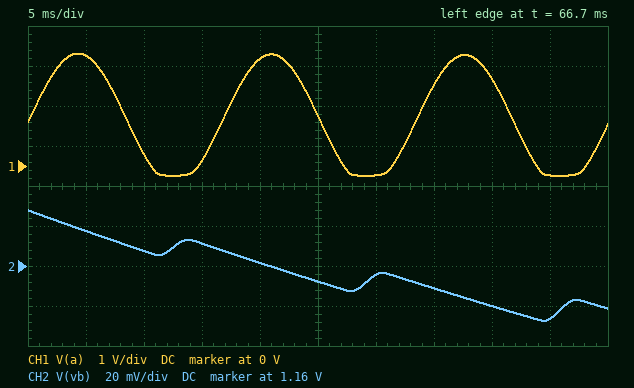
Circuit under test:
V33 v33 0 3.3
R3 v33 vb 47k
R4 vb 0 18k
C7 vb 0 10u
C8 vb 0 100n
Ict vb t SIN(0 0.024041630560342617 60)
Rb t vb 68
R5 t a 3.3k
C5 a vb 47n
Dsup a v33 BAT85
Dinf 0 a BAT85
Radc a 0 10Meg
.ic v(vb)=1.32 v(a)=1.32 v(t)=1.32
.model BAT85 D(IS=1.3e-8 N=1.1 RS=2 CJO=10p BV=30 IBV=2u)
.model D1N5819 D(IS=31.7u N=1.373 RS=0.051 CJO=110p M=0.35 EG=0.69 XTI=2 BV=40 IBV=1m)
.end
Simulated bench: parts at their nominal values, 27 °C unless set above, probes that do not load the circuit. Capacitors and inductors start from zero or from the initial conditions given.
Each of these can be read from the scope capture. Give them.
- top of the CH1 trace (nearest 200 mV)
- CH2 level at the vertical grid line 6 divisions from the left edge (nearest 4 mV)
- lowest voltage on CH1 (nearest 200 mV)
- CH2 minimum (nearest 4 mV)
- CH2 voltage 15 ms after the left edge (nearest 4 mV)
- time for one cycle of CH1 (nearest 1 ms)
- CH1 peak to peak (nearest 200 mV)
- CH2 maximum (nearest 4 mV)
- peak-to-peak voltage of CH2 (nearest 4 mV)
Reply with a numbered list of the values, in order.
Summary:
1. 2.8 V
2. 1.156 V
3. -200 mV
4. 1.132 V
5. 1.172 V
6. 17 ms
7. 3.0 V
8. 1.188 V
9. 56 mV
